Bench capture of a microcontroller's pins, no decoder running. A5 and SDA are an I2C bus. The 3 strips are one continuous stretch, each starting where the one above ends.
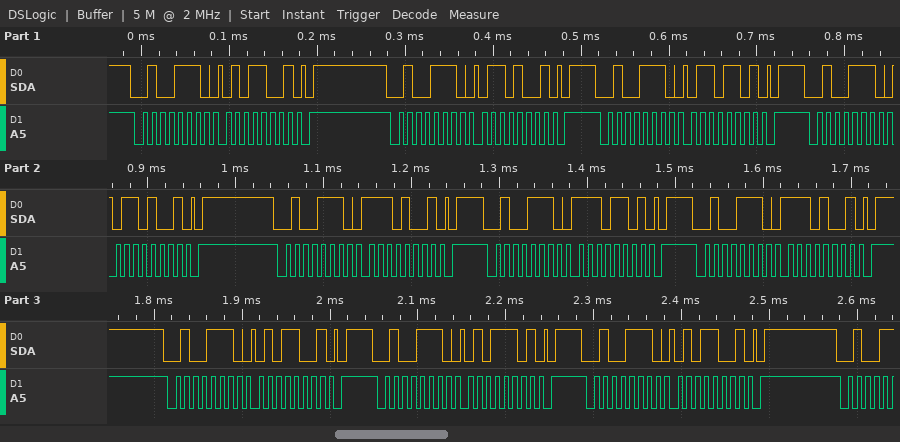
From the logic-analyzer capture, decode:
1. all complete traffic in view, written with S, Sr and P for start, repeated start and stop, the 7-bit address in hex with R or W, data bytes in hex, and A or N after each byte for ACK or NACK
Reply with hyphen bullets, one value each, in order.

- S 27W A 59 A P S 27W A 69 A P S 27W A 6D A P S 27W A 69 A P S 27W A E9 A P S 27W A ED A P S 27W A E9 A P S 27W A 59 A P S 27W A 5D A P S 27W A 59 A P
